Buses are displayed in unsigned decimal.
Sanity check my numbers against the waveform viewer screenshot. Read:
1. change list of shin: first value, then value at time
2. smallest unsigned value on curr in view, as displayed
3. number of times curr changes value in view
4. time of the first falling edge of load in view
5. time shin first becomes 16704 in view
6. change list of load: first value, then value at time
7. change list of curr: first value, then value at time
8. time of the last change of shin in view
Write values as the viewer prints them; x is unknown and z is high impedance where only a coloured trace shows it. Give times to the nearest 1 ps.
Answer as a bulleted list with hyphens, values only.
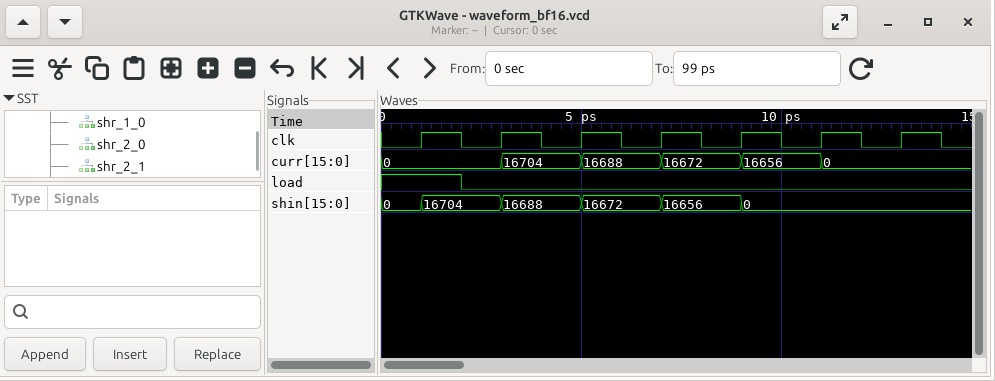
- 0, 16704 at 1 ps, 16688 at 3 ps, 16672 at 5 ps, 16656 at 7 ps, 0 at 9 ps
- 0
- 5
- 2 ps
- 1 ps
- 1, 0 at 2 ps
- 0, 16704 at 3 ps, 16688 at 5 ps, 16672 at 7 ps, 16656 at 9 ps, 0 at 11 ps
- 9 ps
